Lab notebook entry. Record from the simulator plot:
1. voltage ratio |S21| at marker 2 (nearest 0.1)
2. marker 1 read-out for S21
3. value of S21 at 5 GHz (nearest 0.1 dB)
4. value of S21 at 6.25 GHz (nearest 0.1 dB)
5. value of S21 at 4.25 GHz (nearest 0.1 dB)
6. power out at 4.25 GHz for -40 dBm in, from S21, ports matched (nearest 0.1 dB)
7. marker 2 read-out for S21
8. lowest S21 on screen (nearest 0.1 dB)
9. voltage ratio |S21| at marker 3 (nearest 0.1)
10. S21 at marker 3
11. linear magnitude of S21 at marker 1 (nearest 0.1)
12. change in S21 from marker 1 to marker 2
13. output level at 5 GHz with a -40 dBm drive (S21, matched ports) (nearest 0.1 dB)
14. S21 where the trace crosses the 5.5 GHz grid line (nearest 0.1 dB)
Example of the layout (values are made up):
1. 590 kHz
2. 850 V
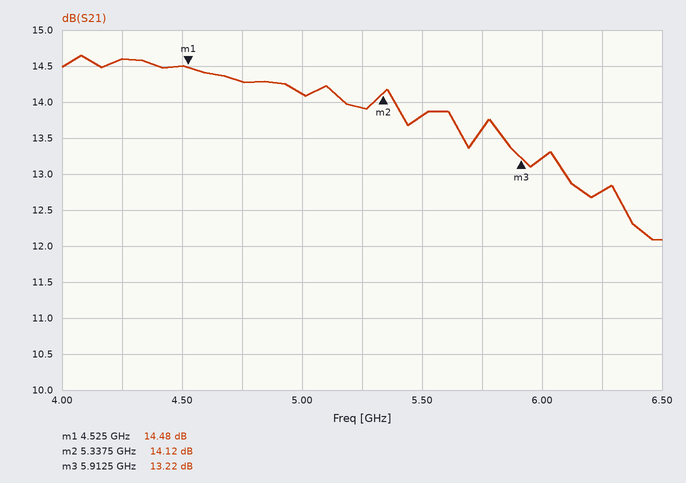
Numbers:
1. 5.1
2. 14.48 dB
3. 14.1 dB
4. 12.8 dB
5. 14.6 dB
6. -25.4 dBm
7. 14.12 dB
8. 12.1 dB
9. 4.6
10. 13.22 dB
11. 5.3
12. -0.36 dB
13. -25.9 dBm
14. 13.8 dB
